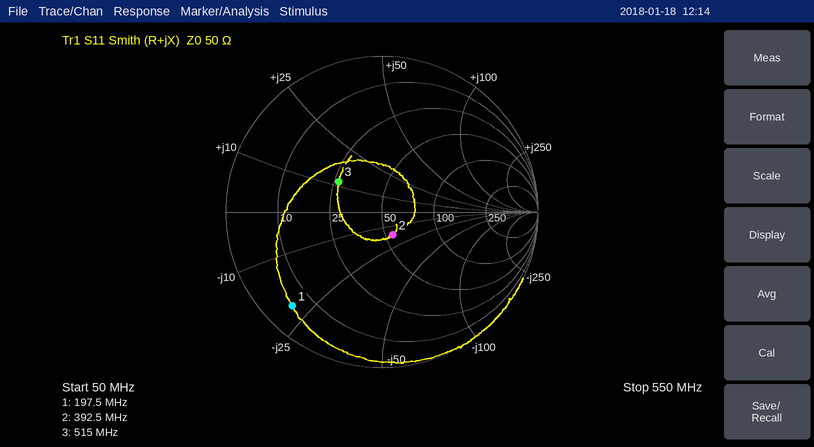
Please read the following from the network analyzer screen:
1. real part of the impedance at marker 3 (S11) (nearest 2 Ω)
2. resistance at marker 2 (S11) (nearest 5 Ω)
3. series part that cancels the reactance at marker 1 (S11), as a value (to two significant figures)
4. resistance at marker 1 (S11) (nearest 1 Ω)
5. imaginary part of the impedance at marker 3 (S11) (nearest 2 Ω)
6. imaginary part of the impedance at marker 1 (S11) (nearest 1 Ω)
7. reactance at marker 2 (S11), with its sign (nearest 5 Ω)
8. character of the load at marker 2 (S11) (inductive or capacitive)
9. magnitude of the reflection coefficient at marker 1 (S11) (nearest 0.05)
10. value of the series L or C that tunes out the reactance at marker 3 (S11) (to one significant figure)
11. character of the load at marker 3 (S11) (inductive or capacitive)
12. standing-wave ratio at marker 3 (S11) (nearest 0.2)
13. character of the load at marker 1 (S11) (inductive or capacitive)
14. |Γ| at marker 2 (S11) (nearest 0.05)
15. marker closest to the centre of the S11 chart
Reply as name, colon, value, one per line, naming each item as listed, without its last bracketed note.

real part of the impedance at marker 3 (S11): 26 Ω
resistance at marker 2 (S11): 55 Ω
series part that cancels the reactance at marker 1 (S11), as a value: 17 nH
resistance at marker 1 (S11): 5 Ω
imaginary part of the impedance at marker 3 (S11): +12 Ω
imaginary part of the impedance at marker 1 (S11): -21 Ω
reactance at marker 2 (S11), with its sign: -15 Ω
character of the load at marker 2 (S11): capacitive
magnitude of the reflection coefficient at marker 1 (S11): 0.85
value of the series L or C that tunes out the reactance at marker 3 (S11): 30 pF
character of the load at marker 3 (S11): inductive
standing-wave ratio at marker 3 (S11): 2.0
character of the load at marker 1 (S11): capacitive
|Γ| at marker 2 (S11): 0.15
marker closest to the centre of the S11 chart: marker 2
